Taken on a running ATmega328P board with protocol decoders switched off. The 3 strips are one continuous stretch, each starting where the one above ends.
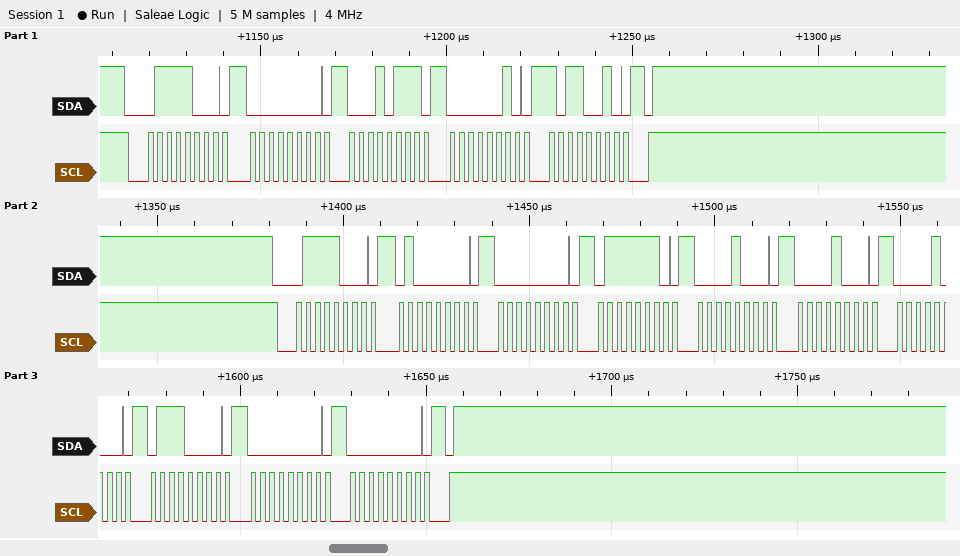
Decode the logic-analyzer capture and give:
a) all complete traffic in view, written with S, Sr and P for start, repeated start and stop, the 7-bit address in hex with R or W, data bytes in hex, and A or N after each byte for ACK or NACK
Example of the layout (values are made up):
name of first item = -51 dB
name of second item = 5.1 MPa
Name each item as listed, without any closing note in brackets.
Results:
all complete traffic in view, written with S, Sr and P for start, repeated start and stop, the 7-bit address in hex with R or W, data bytes in hex, and A or N after each byte for ACK or NACK = S 3CW A 00 A 17 A 02 A B2 A P S 3CW A 40 A 00 A 7E A 08 A 08 A 08 A 70 A 00 A 00 A P
